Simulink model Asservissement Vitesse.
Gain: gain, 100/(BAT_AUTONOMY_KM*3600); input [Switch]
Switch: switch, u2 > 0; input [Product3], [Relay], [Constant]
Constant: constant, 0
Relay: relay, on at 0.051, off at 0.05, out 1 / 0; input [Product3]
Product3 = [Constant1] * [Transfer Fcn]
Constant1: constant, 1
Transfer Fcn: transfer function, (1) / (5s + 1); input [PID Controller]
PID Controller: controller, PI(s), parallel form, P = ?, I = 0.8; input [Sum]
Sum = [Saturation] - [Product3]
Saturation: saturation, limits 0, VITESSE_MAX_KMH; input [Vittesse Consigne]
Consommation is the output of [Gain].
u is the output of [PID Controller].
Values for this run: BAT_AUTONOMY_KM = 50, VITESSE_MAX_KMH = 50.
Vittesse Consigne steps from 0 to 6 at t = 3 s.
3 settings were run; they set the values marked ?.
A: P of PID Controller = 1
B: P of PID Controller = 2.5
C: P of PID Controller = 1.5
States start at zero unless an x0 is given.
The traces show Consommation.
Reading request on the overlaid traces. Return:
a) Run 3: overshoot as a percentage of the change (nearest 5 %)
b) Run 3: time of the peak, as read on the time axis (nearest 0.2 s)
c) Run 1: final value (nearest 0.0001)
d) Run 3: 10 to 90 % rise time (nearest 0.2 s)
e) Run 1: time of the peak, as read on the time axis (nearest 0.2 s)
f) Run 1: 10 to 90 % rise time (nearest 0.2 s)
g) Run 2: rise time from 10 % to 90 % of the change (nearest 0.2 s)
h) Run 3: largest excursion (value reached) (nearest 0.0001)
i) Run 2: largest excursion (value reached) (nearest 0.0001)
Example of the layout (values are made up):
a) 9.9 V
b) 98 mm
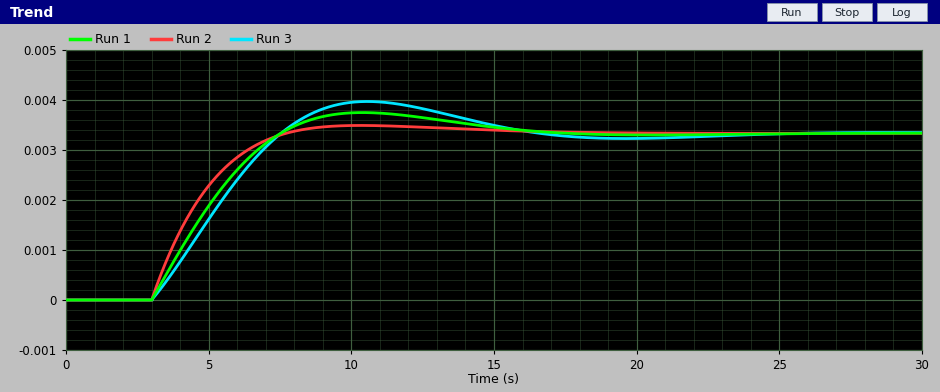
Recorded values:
a) 20 %
b) 10.6 s
c) 0.0033
d) 3.4 s
e) 10.4 s
f) 3.4 s
g) 3.2 s
h) 0.0040
i) 0.0035
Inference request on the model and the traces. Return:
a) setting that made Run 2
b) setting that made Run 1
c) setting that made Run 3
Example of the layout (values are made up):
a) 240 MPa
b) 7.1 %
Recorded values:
a) B
b) C
c) A
